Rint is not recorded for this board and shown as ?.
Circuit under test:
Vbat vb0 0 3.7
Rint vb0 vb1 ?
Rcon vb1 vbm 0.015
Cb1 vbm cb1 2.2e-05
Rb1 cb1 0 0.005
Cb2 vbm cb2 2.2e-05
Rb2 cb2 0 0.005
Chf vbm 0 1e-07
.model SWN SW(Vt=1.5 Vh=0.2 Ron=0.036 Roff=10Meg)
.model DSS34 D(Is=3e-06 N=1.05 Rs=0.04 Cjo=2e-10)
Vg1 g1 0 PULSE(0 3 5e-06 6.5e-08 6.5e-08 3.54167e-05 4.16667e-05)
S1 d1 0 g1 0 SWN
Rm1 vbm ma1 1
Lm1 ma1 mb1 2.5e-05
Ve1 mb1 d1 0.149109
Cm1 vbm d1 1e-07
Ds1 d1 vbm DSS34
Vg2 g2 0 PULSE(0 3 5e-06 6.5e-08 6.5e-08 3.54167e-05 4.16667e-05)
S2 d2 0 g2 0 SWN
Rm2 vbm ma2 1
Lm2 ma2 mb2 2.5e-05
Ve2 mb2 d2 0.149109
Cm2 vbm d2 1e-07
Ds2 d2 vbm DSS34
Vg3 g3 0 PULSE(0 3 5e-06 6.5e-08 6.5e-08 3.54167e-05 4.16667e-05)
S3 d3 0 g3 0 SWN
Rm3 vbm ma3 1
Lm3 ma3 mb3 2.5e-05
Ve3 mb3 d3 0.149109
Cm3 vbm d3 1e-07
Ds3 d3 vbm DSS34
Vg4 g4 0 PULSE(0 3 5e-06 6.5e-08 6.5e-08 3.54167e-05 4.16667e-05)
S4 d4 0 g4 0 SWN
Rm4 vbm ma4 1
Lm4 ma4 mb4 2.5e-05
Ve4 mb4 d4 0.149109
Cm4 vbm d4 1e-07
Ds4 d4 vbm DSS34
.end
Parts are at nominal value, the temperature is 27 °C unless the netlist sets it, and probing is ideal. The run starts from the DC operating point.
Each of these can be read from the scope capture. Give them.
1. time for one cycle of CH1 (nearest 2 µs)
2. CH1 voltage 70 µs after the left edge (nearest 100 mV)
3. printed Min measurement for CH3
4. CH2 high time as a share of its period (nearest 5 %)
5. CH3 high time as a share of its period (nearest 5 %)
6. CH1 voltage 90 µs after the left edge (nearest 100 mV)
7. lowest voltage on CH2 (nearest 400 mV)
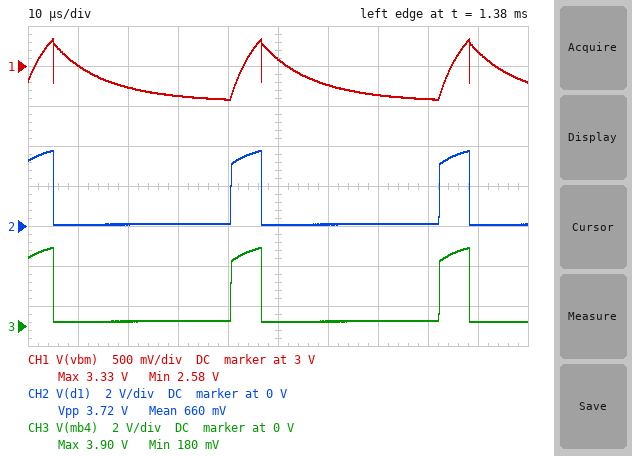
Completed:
42 µs
2.6 V
180 mV
15 %
15 %
3.2 V
0 V
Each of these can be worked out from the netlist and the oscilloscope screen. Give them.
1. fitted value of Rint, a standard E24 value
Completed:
0.11 Ω
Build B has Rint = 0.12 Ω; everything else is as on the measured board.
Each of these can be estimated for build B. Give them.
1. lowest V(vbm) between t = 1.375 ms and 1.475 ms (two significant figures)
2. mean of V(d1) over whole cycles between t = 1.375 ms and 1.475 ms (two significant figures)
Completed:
2.5 V
570 mV
